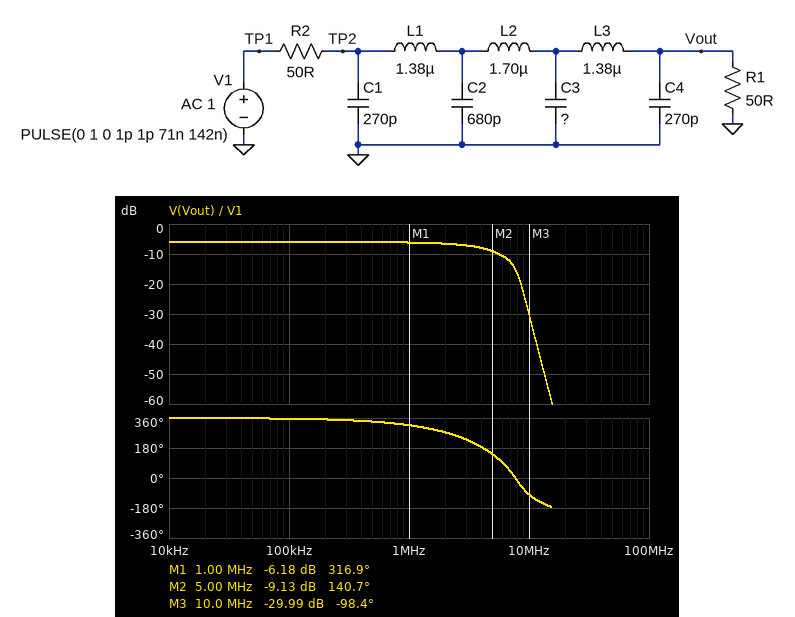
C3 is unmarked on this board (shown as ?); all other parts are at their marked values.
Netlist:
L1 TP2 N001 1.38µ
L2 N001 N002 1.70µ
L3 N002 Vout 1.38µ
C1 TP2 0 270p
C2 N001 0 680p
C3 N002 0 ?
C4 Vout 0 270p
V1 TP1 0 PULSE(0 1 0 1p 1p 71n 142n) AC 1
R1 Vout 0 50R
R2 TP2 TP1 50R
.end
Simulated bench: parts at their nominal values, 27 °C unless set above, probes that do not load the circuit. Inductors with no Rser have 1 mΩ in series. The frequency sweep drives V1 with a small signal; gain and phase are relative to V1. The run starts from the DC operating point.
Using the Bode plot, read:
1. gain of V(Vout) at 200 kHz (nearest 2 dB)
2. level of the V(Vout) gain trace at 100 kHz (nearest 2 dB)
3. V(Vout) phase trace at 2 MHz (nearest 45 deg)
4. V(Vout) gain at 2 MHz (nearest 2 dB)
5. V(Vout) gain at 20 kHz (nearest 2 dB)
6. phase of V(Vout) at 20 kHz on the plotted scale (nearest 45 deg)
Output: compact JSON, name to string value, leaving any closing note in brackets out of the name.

{"gain of V(Vout) at 200 kHz": "-6 dB", "level of the V(Vout) gain trace at 100 kHz": "-6 dB", "V(Vout) phase trace at 2 MHz": "270 deg", "V(Vout) gain at 2 MHz": "-6 dB", "V(Vout) gain at 20 kHz": "-6 dB", "phase of V(Vout) at 20 kHz on the plotted scale": "360 deg"}
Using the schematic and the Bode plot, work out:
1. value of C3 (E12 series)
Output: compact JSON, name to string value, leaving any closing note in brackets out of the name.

{"value of C3": "1.8 nF"}
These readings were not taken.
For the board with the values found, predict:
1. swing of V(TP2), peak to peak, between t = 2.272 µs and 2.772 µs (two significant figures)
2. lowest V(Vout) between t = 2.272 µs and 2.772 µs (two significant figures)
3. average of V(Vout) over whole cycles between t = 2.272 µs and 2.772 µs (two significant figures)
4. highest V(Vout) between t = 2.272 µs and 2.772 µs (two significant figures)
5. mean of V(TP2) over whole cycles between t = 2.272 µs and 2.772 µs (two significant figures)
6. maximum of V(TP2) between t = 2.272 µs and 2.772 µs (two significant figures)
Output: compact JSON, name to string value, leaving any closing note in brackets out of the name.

{"swing of V(TP2), peak to peak, between t = 2.272 µs and 2.772 µs": "680 mV", "lowest V(Vout) between t = 2.272 µs and 2.772 µs": "100 mV", "average of V(Vout) over whole cycles between t = 2.272 µs and 2.772 µs": "250 mV", "highest V(Vout) between t = 2.272 µs and 2.772 µs": "400 mV", "mean of V(TP2) over whole cycles between t = 2.272 µs and 2.772 µs": "250 mV", "maximum of V(TP2) between t = 2.272 µs and 2.772 µs": "590 mV"}
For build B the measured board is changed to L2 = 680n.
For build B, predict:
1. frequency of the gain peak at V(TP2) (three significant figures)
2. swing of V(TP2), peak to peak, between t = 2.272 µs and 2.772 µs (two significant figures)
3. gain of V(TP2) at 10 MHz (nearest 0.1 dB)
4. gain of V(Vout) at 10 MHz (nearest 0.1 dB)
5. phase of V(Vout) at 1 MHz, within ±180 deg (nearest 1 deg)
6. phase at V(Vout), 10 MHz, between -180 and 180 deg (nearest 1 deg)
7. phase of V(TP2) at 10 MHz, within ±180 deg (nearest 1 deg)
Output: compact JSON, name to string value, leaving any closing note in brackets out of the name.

{"frequency of the gain peak at V(TP2)": "11.3 MHz", "swing of V(TP2), peak to peak, between t = 2.272 µs and 2.772 µs": "1.2 V", "gain of V(TP2) at 10 MHz": "-18.1 dB", "gain of V(Vout) at 10 MHz": "-11.2 dB", "phase of V(Vout) at 1 MHz, within ±180 deg": "-39 deg", "phase at V(Vout), 10 MHz, between -180 and 180 deg": "-17 deg", "phase of V(TP2) at 10 MHz, within ±180 deg": "43 deg"}
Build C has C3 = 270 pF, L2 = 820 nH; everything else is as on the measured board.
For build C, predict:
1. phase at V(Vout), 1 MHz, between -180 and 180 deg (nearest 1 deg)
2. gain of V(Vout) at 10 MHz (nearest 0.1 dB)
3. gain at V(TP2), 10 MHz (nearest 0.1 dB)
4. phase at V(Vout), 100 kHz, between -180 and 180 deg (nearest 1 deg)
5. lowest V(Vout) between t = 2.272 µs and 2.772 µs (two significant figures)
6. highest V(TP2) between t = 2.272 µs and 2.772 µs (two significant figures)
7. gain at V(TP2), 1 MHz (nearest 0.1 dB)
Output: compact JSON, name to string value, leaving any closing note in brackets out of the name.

{"phase at V(Vout), 1 MHz, between -180 and 180 deg": "-26 deg", "gain of V(Vout) at 10 MHz": "-13.6 dB", "gain at V(TP2), 10 MHz": "-0.4 dB", "phase at V(Vout), 100 kHz, between -180 and 180 deg": "-3 deg", "lowest V(Vout) between t = 2.272 µs and 2.772 µs": "-33 mV", "highest V(TP2) between t = 2.272 µs and 2.772 µs": "660 mV", "gain at V(TP2), 1 MHz": "-6.0 dB"}
